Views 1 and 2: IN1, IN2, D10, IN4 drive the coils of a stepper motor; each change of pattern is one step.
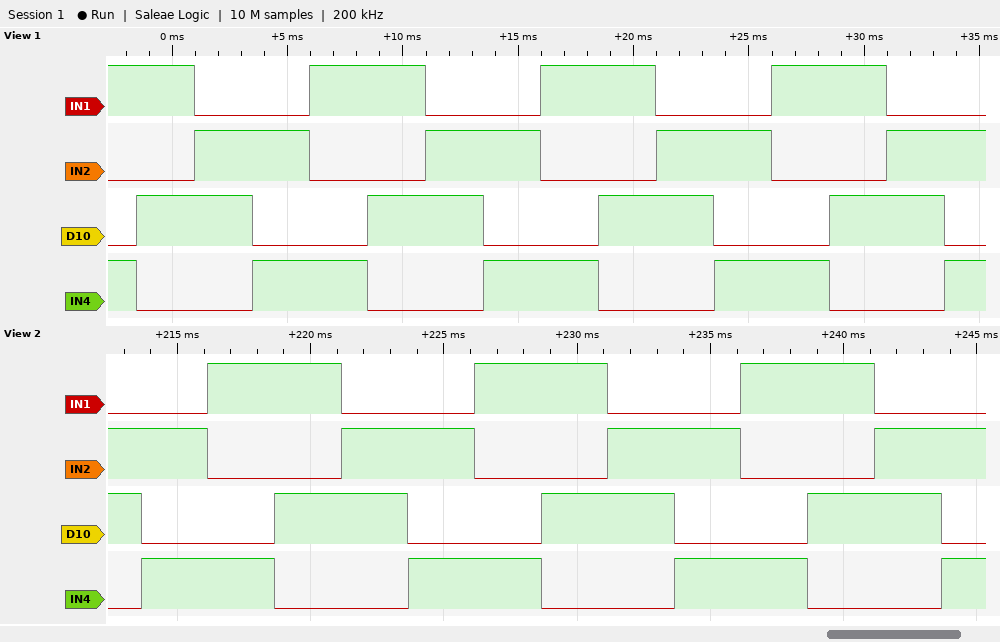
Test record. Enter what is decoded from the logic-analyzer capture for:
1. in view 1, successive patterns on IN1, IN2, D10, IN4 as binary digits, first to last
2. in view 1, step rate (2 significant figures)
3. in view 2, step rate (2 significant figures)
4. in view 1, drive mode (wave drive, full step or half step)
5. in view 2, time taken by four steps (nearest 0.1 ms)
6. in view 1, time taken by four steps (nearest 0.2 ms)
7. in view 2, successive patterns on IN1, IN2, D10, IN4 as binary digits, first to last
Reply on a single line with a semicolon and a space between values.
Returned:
1001 1010 0110 0101 1001 1010 0110 0101 1001 1010 0110 0101 1001 1010 0110 0101; 400 steps/s; 400 steps/s; full step; 10.0 ms; 10.0 ms; 0110 0101 1001 1010 0110 0101 1001 1010 0110 0101 1001 1010 0110 0101
